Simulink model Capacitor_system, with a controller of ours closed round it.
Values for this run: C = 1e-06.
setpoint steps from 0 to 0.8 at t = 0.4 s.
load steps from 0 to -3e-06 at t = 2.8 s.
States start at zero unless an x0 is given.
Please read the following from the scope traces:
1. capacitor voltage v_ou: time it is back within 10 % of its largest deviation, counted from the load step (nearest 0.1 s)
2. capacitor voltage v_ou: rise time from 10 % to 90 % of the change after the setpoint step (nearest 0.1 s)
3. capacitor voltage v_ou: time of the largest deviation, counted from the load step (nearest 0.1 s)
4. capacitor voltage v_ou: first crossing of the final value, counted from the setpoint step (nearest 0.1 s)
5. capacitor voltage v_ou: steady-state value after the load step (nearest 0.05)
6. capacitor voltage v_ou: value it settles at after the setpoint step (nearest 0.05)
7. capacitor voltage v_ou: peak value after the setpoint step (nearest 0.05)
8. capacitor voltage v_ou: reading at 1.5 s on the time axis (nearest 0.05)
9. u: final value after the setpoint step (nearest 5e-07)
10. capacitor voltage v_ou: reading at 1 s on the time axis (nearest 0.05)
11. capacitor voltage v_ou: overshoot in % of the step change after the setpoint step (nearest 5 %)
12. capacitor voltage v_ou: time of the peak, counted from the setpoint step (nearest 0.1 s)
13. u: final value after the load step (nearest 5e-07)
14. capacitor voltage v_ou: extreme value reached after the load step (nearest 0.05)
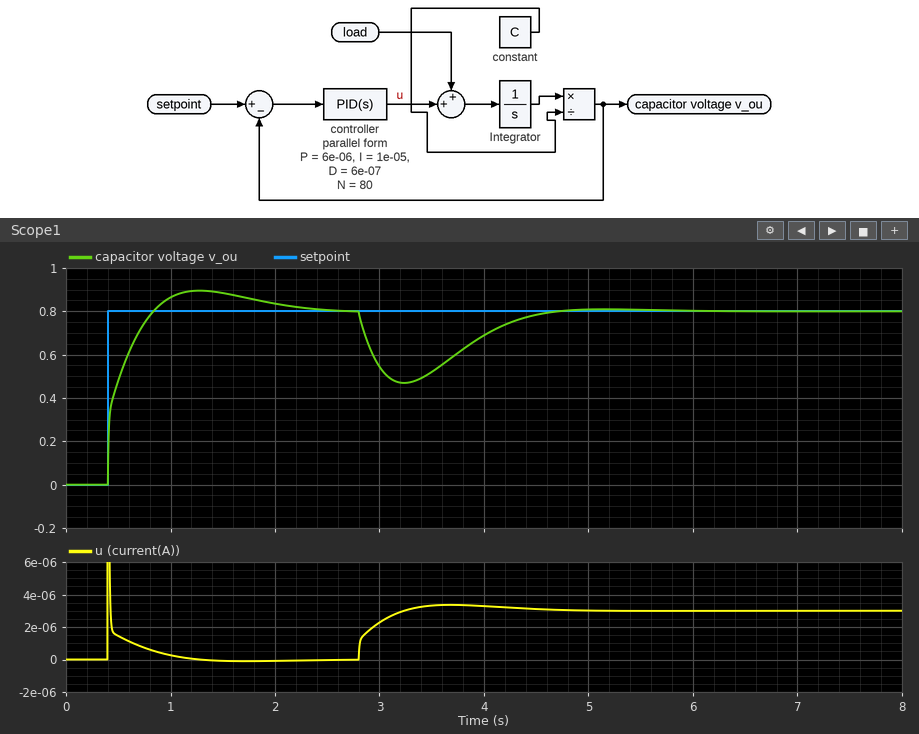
1.6 s
0.3 s
0.4 s
0.4 s
0.80
0.80
0.90
0.90
0.0000000
0.85
10 %
0.9 s
0.0000030
0.45
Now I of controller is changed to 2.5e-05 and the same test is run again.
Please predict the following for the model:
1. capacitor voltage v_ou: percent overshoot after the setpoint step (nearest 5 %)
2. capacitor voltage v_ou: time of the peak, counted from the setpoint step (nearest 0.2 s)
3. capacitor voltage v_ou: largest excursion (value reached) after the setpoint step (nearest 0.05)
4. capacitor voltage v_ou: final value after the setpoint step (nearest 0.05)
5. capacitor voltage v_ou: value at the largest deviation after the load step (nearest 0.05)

20 %
0.6 s
0.95
0.80
0.55
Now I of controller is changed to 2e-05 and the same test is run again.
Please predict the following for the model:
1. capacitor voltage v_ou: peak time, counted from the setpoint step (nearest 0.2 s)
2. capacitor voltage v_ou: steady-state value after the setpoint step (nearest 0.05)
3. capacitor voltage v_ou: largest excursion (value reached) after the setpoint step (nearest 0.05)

0.6 s
0.80
0.95
